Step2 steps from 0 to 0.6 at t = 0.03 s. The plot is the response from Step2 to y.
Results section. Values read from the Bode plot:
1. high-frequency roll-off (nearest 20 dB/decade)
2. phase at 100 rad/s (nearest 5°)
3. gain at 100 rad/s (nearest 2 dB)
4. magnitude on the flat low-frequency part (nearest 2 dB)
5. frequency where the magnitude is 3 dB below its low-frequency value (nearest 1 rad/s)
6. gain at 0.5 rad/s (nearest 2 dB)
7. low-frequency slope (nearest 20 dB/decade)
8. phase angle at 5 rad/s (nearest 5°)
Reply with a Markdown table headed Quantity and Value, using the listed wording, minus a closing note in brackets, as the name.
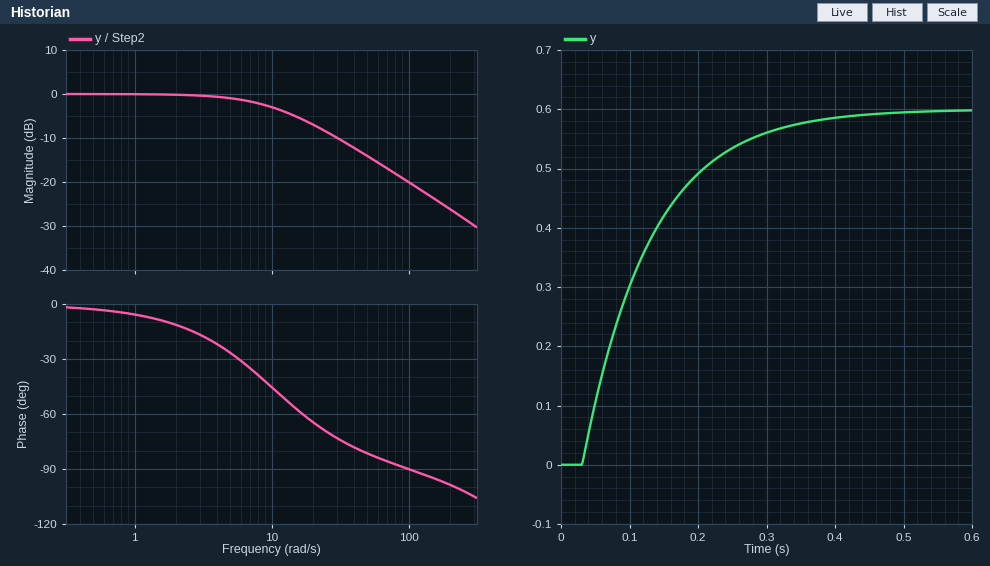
| Quantity | Value |
|---|---|
| high-frequency roll-off | -20 dB/decade |
| phase at 100 rad/s | -90° |
| gain at 100 rad/s | -20 dB |
| magnitude on the flat low-frequency part | 0 dB |
| frequency where the magnitude is 3 dB below its low-frequency value | 10 rad/s |
| gain at 0.5 rad/s | 0 dB |
| low-frequency slope | 0 dB/decade |
| phase angle at 5 rad/s | -25° |
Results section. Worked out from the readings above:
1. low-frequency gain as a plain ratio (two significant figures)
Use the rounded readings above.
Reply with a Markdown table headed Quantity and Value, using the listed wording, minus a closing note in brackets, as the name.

| Quantity | Value |
|---|---|
| low-frequency gain as a plain ratio | 1.0 |
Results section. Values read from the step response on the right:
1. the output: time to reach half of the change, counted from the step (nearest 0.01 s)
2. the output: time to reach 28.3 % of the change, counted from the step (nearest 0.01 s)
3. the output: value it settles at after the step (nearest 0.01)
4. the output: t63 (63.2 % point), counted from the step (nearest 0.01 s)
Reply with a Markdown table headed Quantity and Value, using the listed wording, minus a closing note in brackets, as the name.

| Quantity | Value |
|---|---|
| the output: time to reach half of the change, counted from the step | 0.07 s |
| the output: time to reach 28.3 % of the change, counted from the step | 0.03 s |
| the output: value it settles at after the step | 0.60 |
| the output: t63 (63.2 % point), counted from the step | 0.10 s |
